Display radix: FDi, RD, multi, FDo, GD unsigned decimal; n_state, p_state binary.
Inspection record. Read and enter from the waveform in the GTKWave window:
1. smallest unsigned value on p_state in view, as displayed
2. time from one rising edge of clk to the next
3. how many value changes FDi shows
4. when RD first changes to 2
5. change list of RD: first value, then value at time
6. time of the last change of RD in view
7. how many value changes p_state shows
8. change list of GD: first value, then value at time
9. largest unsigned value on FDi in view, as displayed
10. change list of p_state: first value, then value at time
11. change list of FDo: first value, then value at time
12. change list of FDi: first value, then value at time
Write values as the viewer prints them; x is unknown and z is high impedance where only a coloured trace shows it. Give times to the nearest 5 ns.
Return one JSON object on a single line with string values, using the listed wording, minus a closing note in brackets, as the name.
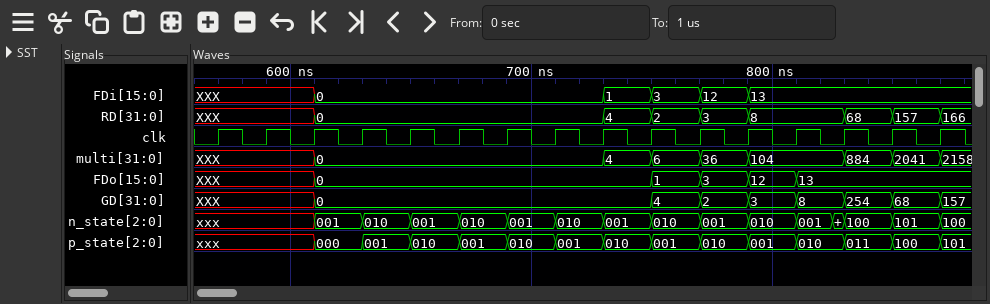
{"smallest unsigned value on p_state in view, as displayed": "000", "time from one rising edge of clk to the next": "20 ns", "how many value changes FDi shows": "5", "when RD first changes to 2": "750 ns", "change list of RD: first value, then value at time": "XXX, 0 at 610 ns, 4 at 730 ns, 2 at 750 ns, 3 at 770 ns, 8 at 790 ns, 68 at 830 ns, 157 at 850 ns, 166 at 870 ns", "time of the last change of RD in view": "870 ns", "how many value changes p_state shows": "14", "change list of GD: first value, then value at time": "XXX, 0 at 610 ns, 4 at 750 ns, 2 at 770 ns, 3 at 790 ns, 8 at 810 ns, 254 at 830 ns, 68 at 850 ns, 157 at 870 ns", "largest unsigned value on FDi in view, as displayed": "13", "change list of p_state: first value, then value at time": "xxx, 000 at 610 ns, 001 at 630 ns, 010 at 650 ns, 001 at 670 ns, 010 at 690 ns, 001 at 710 ns, 010 at 730 ns, 001 at 750 ns, 010 at 770 ns, 001 at 790 ns, 010 at 810 ns, 011 at 830 ns, 100 at 850 ns, 101 at 870 ns", "change list of FDo: first value, then value at time": "XXX, 0 at 610 ns, 1 at 750 ns, 3 at 770 ns, 12 at 790 ns, 13 at 810 ns", "change list of FDi: first value, then value at time": "XXX, 0 at 610 ns, 1 at 730 ns, 3 at 750 ns, 12 at 770 ns, 13 at 790 ns"}
